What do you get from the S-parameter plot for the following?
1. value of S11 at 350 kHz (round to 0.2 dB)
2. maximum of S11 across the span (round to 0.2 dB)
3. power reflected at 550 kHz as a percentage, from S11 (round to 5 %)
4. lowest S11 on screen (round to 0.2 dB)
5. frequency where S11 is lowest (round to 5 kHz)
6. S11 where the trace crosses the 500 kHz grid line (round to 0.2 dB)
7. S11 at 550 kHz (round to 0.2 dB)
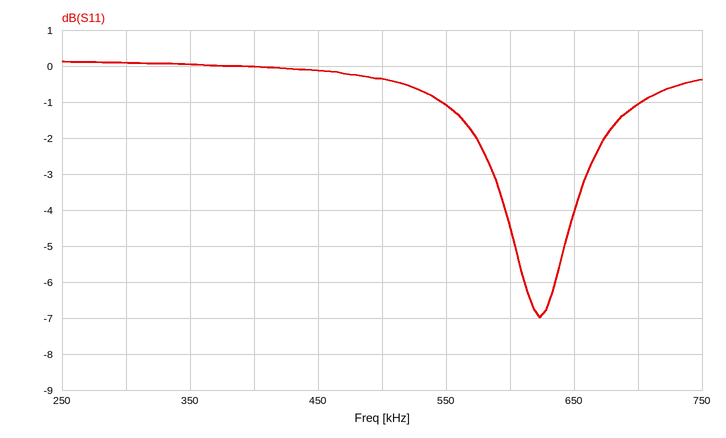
0.0 dB
0.2 dB
80 %
-7.0 dB
625 kHz
-0.4 dB
-1.0 dB
